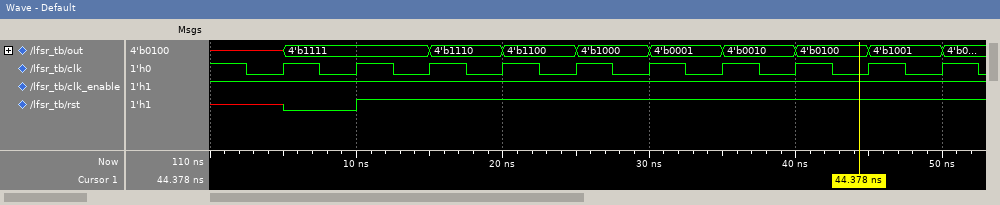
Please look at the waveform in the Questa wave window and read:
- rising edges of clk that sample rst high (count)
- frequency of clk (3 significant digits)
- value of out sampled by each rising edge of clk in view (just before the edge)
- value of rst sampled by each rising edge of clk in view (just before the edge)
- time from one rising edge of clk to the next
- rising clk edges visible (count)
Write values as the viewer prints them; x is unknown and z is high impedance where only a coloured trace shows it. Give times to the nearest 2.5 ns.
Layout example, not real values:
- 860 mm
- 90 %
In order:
- 8
- 200 MHz
- x, 4'b1111, 4'b1111, 4'b1110, 4'b1100, 4'b1000, 4'b0001, 4'b0010, 4'b0100, 4'b1001
- x 0 1 1 1 1 1 1 1 1
- 5 ns
- 10
